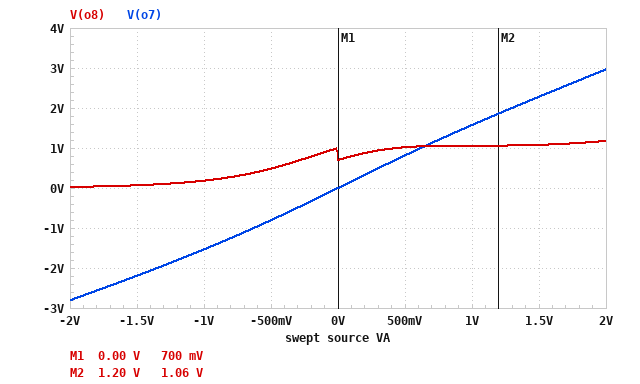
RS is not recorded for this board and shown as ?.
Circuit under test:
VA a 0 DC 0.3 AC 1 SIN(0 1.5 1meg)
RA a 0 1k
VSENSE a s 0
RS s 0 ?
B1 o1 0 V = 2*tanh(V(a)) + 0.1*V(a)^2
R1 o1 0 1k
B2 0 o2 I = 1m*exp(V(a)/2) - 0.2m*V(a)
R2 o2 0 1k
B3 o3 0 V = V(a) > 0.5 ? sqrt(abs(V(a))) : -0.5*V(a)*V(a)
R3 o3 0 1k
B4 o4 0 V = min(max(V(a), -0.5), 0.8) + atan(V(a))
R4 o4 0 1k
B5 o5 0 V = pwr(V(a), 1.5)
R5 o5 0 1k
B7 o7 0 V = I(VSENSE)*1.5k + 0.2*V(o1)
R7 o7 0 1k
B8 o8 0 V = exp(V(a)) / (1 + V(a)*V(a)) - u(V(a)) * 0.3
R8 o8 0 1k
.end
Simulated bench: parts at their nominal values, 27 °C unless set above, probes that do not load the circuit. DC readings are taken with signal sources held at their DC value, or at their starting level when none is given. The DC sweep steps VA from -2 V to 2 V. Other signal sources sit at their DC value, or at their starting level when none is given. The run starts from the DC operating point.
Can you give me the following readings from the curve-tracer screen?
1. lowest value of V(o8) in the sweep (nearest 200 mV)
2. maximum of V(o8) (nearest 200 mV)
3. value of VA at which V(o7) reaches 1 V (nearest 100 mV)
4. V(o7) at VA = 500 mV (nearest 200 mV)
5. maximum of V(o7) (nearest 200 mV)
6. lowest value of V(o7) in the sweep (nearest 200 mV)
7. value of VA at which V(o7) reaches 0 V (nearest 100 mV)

0 V
1.2 V
600 mV
800 mV
3.0 V
-2.8 V
0 V
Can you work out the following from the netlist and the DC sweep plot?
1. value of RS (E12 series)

1.2 kΩ
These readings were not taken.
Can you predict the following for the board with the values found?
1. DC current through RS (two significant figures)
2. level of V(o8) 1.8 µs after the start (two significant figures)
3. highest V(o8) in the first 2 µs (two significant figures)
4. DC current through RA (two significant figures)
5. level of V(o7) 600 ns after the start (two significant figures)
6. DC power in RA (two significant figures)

250 µA
79 mV
1.1 V
300 µA
-1.4 V
90 µW
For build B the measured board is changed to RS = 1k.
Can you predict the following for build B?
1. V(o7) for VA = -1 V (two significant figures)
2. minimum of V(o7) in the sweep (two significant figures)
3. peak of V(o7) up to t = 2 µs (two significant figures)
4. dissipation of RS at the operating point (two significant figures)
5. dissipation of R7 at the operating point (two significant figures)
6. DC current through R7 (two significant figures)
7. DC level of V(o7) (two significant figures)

-1.8 V
-3.3 V
2.7 V
90 µW
320 µW
570 µA
570 mV
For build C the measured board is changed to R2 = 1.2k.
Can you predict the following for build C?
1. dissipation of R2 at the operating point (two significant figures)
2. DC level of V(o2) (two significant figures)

1.5 mW
1.3 V
